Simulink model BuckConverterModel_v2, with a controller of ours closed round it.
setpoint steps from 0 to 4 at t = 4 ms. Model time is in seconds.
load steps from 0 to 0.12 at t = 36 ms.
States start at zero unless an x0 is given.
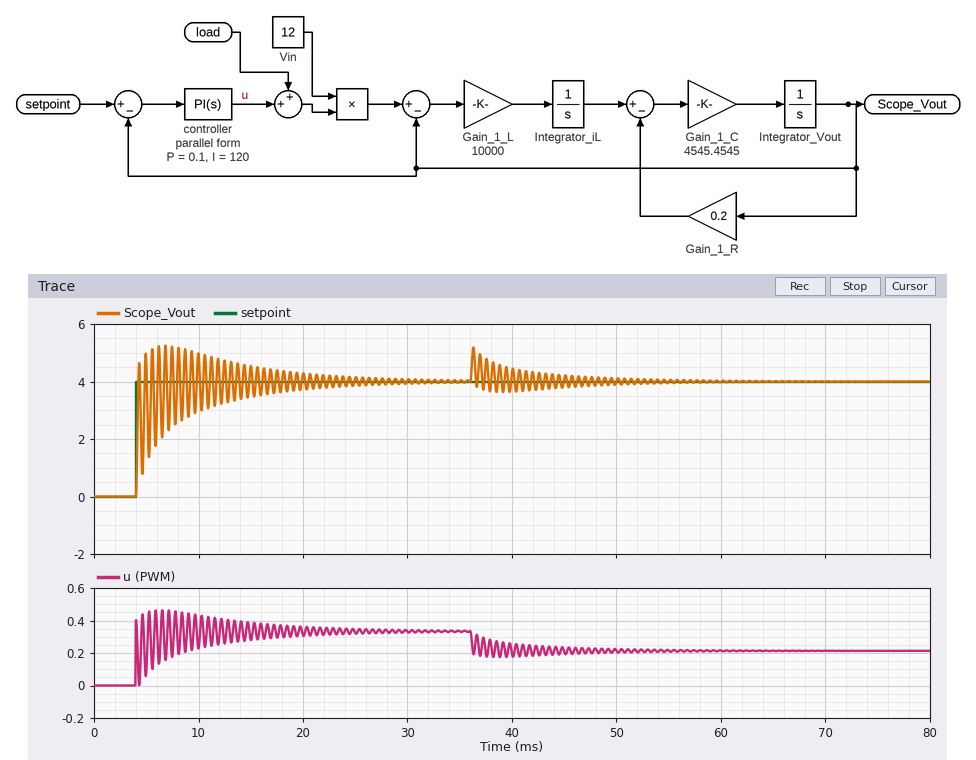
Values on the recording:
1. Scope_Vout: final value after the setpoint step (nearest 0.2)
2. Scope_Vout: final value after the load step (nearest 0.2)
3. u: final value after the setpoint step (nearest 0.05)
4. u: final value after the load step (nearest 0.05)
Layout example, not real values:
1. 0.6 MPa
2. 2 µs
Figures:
1. 4.0
2. 4.0
3. 0.35
4. 0.20
